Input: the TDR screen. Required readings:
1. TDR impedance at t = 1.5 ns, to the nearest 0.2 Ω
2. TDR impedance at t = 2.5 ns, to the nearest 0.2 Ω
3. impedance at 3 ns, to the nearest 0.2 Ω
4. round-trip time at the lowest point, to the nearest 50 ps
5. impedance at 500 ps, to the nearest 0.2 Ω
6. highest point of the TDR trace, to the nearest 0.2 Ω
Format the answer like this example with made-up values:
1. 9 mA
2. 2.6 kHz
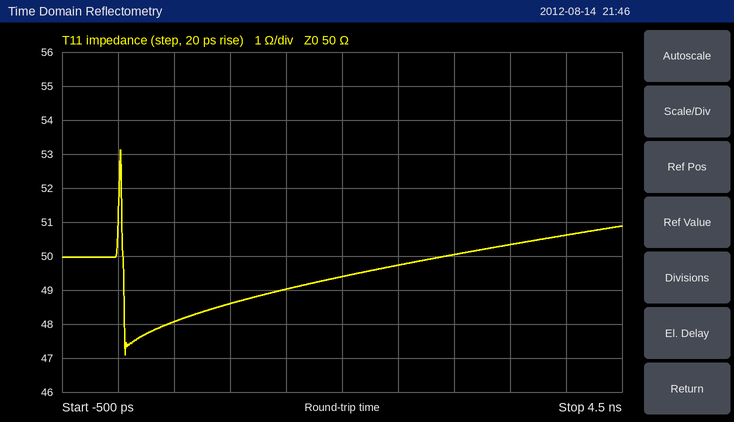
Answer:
1. 49.0 Ω
2. 49.8 Ω
3. 50.0 Ω
4. 50 ps
5. 48.0 Ω
6. 53.2 Ω
